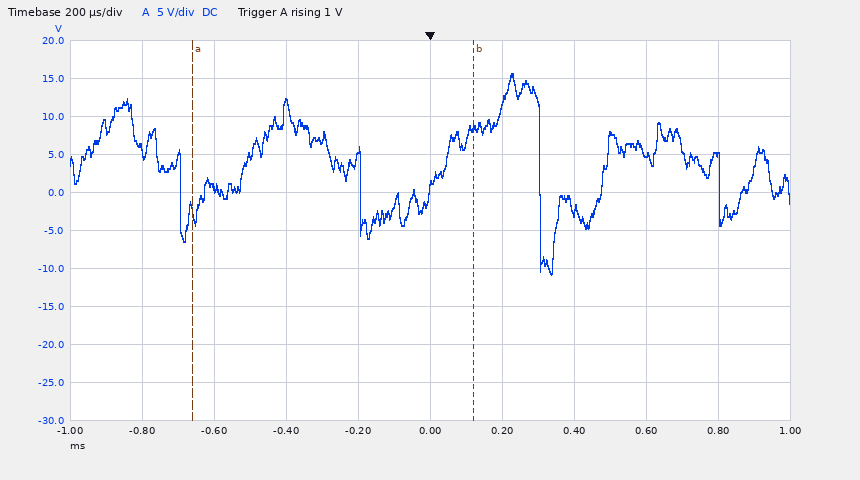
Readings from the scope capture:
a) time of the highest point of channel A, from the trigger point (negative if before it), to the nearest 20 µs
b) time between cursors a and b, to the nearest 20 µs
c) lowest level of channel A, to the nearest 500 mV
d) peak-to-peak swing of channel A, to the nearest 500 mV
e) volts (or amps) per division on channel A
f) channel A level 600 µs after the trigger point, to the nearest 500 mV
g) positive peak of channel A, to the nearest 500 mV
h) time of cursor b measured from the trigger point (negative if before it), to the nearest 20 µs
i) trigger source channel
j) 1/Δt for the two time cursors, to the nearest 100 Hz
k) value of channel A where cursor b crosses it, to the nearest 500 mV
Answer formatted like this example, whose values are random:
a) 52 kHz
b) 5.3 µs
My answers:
a) +220 µs
b) 780 µs
c) -11.0 V
d) 26.5 V
e) 5 V
f) 5.0 V
g) 15.5 V
h) +120 µs
i) channel A
j) 1.3 kHz
k) 8.5 V
